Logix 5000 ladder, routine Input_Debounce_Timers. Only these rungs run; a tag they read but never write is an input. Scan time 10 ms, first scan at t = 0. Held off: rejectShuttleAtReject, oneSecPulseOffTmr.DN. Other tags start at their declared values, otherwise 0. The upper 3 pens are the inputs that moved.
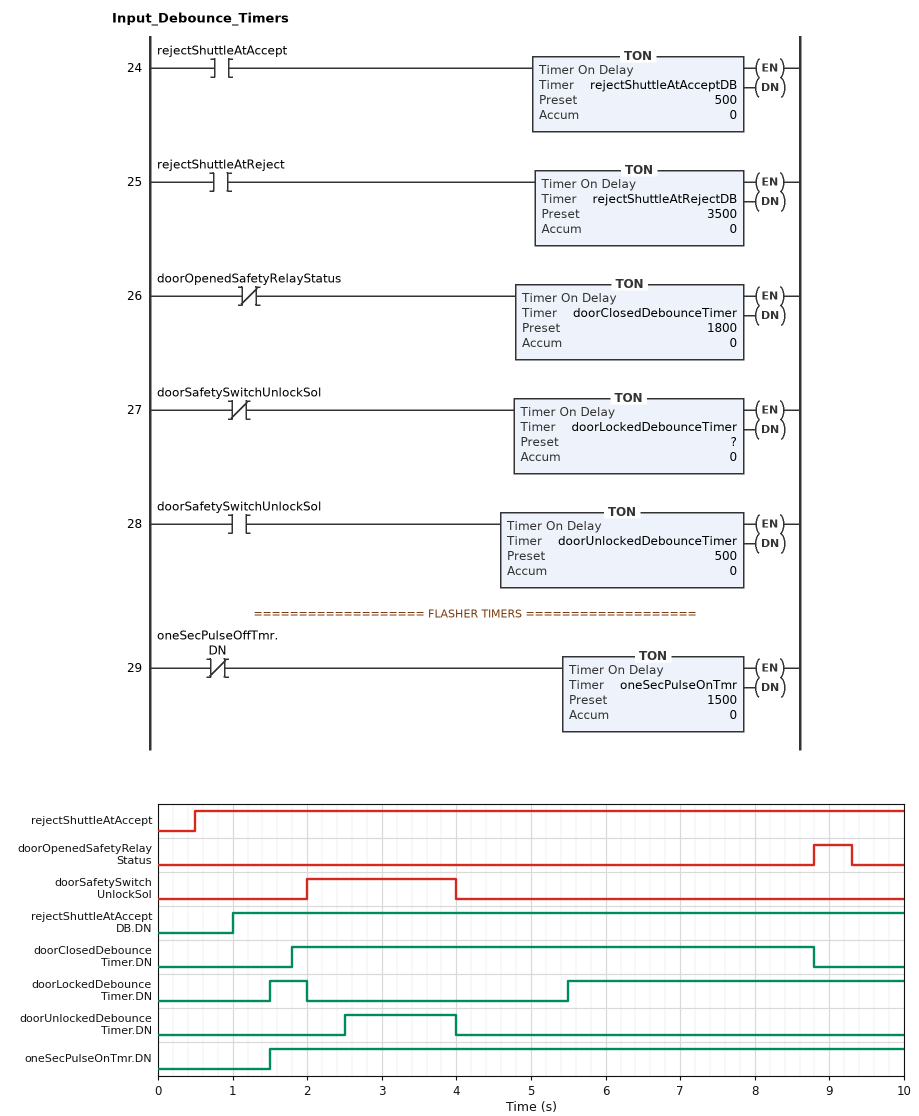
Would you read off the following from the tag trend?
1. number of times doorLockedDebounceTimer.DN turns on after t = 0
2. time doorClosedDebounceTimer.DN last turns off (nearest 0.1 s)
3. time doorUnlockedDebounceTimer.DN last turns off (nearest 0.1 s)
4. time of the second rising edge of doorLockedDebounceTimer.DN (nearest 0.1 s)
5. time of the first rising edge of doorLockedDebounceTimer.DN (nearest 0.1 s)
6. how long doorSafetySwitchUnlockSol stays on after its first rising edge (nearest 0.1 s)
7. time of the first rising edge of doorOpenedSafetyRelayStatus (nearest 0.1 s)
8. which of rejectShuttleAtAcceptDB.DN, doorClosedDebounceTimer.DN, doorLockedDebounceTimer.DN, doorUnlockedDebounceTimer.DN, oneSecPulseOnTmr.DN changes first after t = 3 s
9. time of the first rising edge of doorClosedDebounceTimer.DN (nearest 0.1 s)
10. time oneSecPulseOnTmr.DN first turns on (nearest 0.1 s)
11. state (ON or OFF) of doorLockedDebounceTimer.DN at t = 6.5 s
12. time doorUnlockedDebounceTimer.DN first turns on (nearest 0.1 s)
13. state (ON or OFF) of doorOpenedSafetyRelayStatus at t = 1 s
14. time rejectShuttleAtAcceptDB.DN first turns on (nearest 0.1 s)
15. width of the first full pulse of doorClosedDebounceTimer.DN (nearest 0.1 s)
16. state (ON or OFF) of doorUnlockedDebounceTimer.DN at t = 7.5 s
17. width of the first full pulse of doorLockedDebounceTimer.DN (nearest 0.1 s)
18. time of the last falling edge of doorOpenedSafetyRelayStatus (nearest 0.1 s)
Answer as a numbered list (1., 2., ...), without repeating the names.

1. 2
2. 8.8 s
3. 4.0 s
4. 5.5 s
5. 1.5 s
6. 2.0 s
7. 8.8 s
8. doorUnlockedDebounceTimer.DN
9. 1.8 s
10. 1.5 s
11. ON
12. 2.5 s
13. OFF
14. 1.0 s
15. 7.0 s
16. OFF
17. 0.5 s
18. 9.3 s
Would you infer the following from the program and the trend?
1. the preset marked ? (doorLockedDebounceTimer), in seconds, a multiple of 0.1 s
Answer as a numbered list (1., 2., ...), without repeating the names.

1. 1.5 s
